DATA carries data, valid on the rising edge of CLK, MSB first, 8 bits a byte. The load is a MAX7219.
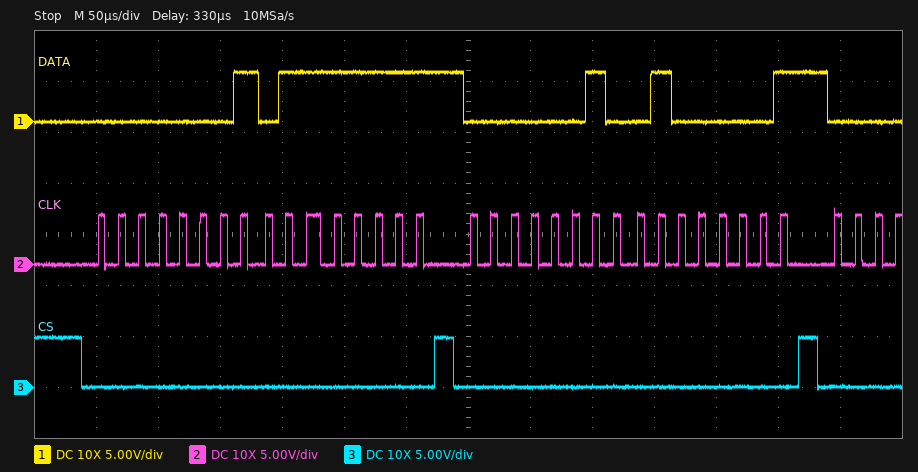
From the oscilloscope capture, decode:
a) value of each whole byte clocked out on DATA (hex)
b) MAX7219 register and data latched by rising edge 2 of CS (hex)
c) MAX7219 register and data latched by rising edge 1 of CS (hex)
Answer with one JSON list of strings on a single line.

["01 7F 02 41", "register 0x2, data 0x41", "register 0x1, data 0x7F"]
